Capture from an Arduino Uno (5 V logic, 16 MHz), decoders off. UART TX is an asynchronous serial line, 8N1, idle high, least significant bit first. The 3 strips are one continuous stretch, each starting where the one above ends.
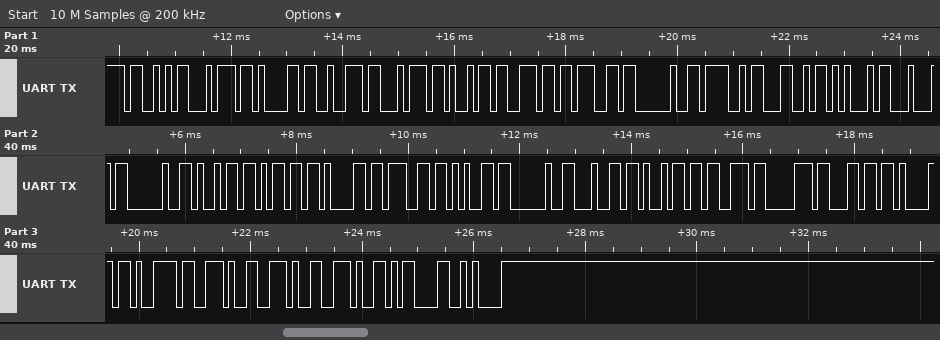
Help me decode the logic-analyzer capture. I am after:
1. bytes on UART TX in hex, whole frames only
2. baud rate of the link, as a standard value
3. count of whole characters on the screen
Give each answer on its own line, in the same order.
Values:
53 74 61 72 74 69 6E 67 20 4F 4C 45 44 20 69 6D 61 67 65 20 64 69 73 70 6C 61 79 2E 2E 2E 0D 0A
9600 baud
32
